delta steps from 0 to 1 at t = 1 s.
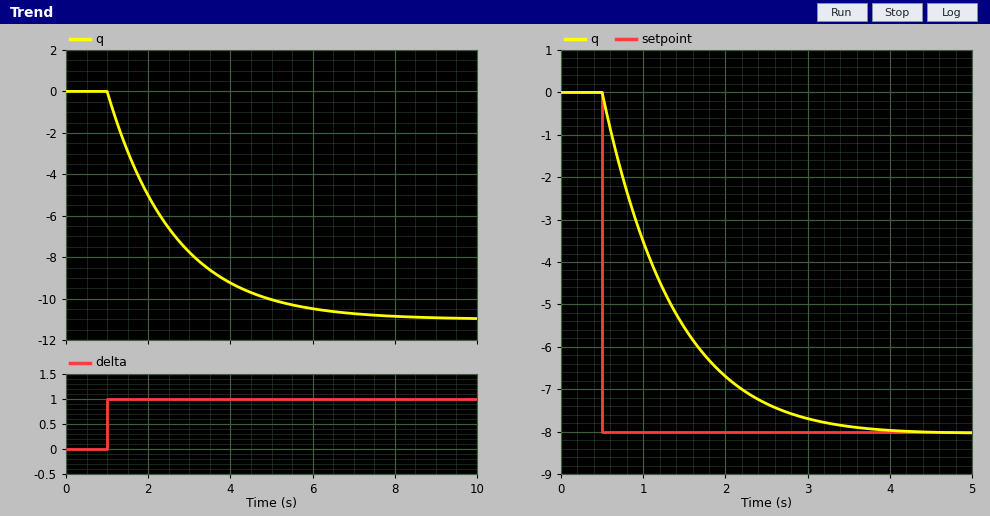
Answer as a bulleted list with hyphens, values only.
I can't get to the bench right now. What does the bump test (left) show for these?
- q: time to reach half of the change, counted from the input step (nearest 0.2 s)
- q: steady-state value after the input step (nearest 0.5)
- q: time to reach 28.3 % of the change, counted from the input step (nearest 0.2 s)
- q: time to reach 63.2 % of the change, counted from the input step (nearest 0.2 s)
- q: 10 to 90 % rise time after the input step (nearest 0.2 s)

- 1.2 s
- -11.0
- 0.6 s
- 1.6 s
- 3.6 s
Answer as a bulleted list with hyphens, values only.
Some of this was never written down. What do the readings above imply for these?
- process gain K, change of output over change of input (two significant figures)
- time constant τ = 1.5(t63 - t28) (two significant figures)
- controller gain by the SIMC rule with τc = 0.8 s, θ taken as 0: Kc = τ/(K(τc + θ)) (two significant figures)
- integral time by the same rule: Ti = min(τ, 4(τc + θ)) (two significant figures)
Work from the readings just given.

- -11
- 1.5 s
- -0.17
- 1.5 s
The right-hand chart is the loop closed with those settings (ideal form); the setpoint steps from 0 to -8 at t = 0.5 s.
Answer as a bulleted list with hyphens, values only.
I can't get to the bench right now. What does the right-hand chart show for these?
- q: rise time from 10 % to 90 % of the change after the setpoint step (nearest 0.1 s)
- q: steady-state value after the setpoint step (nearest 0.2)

- 1.8 s
- -8.0
